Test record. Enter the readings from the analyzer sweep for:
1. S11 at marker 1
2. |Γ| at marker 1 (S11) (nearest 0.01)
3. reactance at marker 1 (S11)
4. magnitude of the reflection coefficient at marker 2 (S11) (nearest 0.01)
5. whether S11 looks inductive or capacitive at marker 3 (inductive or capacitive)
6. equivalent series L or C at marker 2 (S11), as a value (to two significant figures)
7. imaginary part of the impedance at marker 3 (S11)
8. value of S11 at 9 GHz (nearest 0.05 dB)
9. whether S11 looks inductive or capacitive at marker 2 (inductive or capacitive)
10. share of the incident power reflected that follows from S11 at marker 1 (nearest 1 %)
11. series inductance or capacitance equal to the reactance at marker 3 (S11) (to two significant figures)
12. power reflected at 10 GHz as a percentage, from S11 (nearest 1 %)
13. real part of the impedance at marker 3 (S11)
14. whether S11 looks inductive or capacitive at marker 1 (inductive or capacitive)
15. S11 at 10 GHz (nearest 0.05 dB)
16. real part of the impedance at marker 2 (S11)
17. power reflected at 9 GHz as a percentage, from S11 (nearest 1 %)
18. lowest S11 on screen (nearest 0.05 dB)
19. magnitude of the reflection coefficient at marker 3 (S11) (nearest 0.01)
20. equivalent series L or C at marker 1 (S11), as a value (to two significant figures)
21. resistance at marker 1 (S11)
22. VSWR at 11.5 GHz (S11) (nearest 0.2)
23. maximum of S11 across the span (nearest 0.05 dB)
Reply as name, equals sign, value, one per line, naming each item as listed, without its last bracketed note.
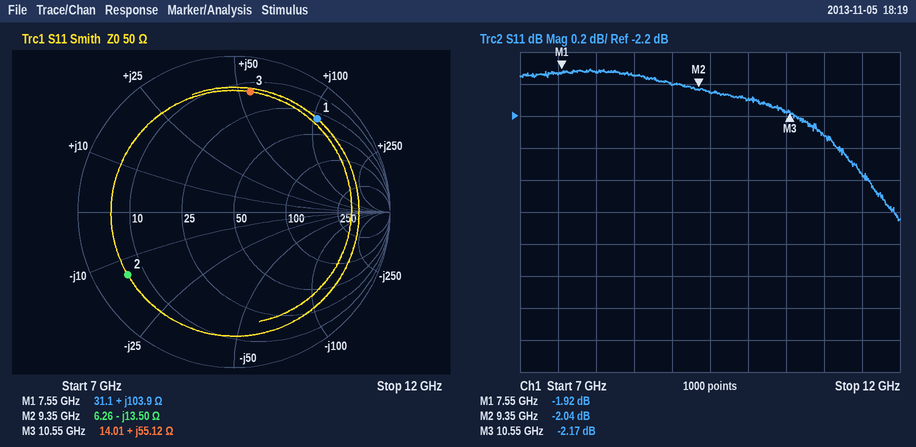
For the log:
S11 at marker 1 = -1.92 dB
|Γ| at marker 1 (S11) = 0.80
reactance at marker 1 = +103.9 Ω
magnitude of the reflection coefficient at marker 2 (S11) = 0.79
whether S11 looks inductive or capacitive at marker 3 = inductive
equivalent series L or C at marker 2 (S11), as a value = 1.3 pF
imaginary part of the impedance at marker 3 = +55.12 Ω
value of S11 at 9 GHz = -2.00 dB
whether S11 looks inductive or capacitive at marker 2 = capacitive
share of the incident power reflected that follows from S11 at marker 1 = 64 %
series inductance or capacitance equal to the reactance at marker 3 (S11) = 830 pH
power reflected at 10 GHz as a percentage, from S11 = 62 %
real part of the impedance at marker 3 = 14.01 Ω
whether S11 looks inductive or capacitive at marker 1 = inductive
S11 at 10 GHz = -2.10 dB
real part of the impedance at marker 2 = 6.26 Ω
power reflected at 9 GHz as a percentage, from S11 = 63 %
lowest S11 on screen = -2.85 dB
magnitude of the reflection coefficient at marker 3 (S11) = 0.78
equivalent series L or C at marker 1 (S11), as a value = 2.2 nH
resistance at marker 1 = 31.1 Ω
VSWR at 11.5 GHz (S11) = 6.8
maximum of S11 across the span = -1.90 dB
